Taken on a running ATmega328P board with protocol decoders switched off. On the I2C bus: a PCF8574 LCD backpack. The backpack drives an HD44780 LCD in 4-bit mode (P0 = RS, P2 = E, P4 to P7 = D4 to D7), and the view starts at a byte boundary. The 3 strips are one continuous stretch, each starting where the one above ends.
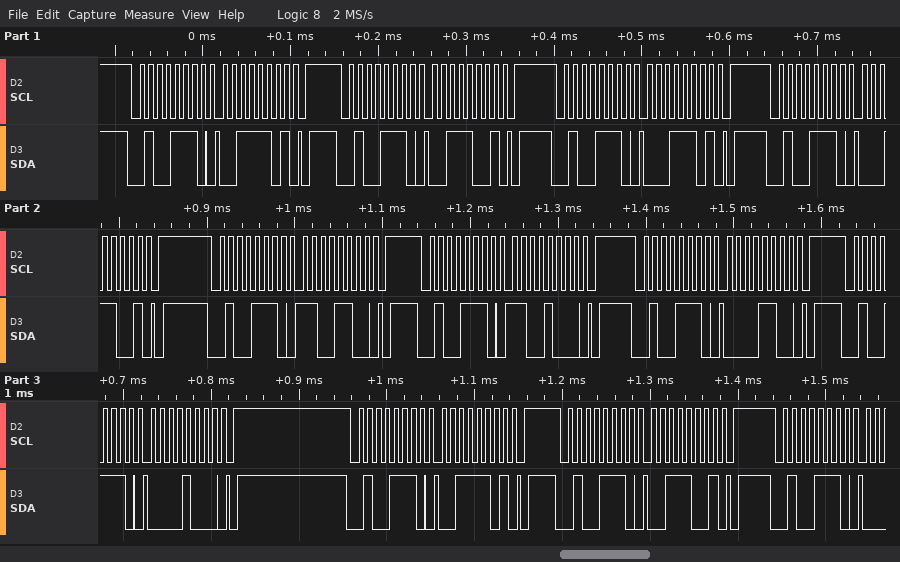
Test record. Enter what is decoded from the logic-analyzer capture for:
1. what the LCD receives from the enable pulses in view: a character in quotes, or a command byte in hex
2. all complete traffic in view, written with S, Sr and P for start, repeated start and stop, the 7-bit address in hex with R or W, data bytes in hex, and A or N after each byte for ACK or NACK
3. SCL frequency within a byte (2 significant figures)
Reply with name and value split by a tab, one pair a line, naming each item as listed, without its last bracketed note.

what the LCD receives from the enable pulses in view: a character in quotes, or a command byte in hex	'1' 0xC0
all complete traffic in view, written with S, Sr and P for start, repeated start and stop, the 7-bit address in hex with R or W, data bytes in hex, and A or N after each byte for ACK or NACK	S 27W A 3D A P S 27W A 39 A P S 27W A 1D A P S 27W A 19 A P S 27W A CC A P S 27W A C8 A P S 27W A 0C A P S 27W A 08 A P S 27W A 3D A P S 27W A 39 A P S 27W A
SCL frequency within a byte	100 kHz
